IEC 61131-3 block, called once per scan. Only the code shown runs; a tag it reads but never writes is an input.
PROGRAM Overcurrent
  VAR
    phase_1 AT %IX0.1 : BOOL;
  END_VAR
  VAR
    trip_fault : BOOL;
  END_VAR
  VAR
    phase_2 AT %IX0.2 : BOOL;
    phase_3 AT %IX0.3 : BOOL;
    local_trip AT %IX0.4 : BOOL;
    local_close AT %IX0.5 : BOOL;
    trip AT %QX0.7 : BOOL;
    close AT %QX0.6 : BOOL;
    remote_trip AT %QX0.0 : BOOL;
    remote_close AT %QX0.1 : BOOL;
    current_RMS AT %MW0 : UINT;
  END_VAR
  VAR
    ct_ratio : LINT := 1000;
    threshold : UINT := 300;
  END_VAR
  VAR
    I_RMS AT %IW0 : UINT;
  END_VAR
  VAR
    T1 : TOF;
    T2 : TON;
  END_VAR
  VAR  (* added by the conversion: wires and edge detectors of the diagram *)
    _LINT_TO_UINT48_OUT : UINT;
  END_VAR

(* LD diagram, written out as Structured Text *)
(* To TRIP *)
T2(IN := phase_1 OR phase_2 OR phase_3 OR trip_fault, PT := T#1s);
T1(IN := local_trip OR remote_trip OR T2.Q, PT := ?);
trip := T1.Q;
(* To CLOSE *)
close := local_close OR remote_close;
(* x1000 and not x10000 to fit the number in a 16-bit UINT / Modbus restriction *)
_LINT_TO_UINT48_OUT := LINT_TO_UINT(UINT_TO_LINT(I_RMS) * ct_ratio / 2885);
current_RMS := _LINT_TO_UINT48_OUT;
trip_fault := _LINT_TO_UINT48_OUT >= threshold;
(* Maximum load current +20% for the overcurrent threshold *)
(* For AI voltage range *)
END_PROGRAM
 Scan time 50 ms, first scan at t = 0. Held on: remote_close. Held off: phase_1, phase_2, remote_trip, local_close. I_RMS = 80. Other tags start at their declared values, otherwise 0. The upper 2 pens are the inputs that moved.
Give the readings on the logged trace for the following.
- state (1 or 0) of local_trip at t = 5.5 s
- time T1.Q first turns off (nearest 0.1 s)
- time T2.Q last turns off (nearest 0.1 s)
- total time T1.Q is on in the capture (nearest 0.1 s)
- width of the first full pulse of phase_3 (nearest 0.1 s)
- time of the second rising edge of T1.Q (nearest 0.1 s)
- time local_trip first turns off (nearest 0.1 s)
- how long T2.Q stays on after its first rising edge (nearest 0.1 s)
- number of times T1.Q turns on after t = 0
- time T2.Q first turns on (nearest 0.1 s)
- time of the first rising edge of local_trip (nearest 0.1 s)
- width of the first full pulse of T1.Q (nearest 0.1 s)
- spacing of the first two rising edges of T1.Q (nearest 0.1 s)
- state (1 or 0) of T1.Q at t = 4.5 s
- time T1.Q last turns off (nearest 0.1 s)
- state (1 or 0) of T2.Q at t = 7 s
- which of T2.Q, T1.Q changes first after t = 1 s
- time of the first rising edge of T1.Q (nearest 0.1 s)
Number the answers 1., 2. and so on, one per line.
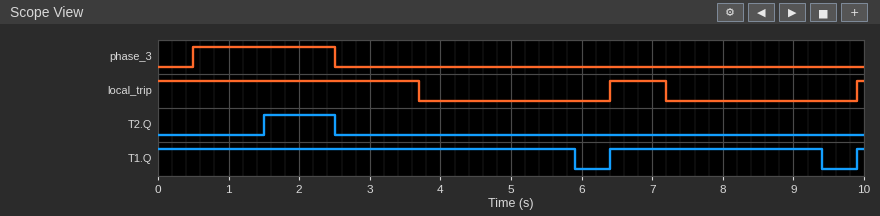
1. 0
2. 5.9 s
3. 2.5 s
4. 9.0 s
5. 2.0 s
6. 9.9 s
7. 3.7 s
8. 1.0 s
9. 2
10. 1.5 s
11. 6.4 s
12. 3.0 s
13. 3.5 s
14. 1
15. 9.4 s
16. 0
17. T2.Q
18. 6.4 s
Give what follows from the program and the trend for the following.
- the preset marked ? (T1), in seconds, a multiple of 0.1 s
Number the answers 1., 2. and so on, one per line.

1. 2.2 s
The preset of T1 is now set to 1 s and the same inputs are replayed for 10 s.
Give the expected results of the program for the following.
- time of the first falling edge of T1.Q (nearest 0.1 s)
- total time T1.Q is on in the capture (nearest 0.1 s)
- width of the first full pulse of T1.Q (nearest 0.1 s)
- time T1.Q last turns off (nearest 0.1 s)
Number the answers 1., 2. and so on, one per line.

1. 4.7 s
2. 6.6 s
3. 1.8 s
4. 8.2 s
